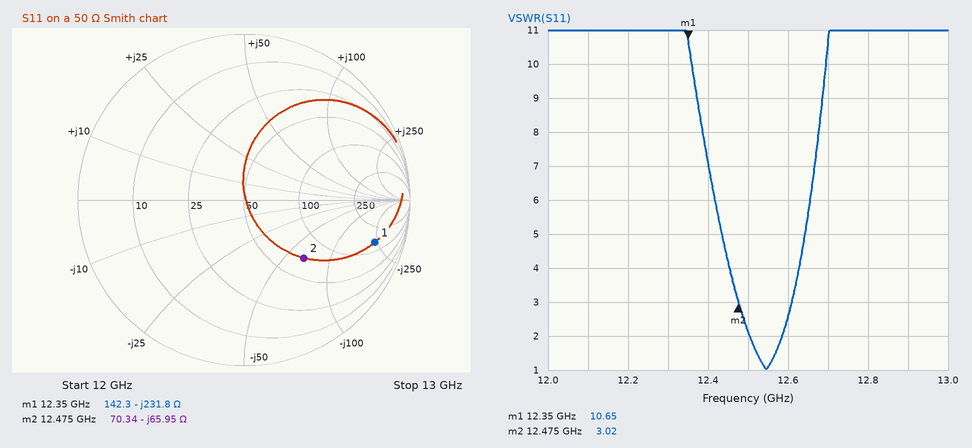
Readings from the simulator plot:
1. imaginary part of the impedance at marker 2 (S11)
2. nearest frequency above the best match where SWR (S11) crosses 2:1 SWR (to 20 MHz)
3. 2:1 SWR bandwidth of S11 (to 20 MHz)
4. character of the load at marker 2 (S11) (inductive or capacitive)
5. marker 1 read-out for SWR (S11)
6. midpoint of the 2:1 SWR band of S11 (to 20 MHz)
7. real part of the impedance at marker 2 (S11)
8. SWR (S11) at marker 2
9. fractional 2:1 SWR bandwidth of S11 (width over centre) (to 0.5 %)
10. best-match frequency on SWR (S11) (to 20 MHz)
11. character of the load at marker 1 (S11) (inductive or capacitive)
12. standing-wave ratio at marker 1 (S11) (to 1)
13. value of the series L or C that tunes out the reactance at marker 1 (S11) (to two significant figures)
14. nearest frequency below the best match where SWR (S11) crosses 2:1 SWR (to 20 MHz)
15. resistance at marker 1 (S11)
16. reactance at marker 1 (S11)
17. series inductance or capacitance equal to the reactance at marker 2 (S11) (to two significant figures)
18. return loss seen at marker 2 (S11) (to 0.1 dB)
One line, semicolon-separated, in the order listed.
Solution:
-65.95 Ω; 12.58 GHz; 80 MHz; capacitive; 10.65; 12.54 GHz; 70.34 Ω; 3.02; 0.5 %; 12.54 GHz; capacitive; 11; 3.0 nH; 12.50 GHz; 142.3 Ω; -231.8 Ω; 190 fF; 6.0 dB
